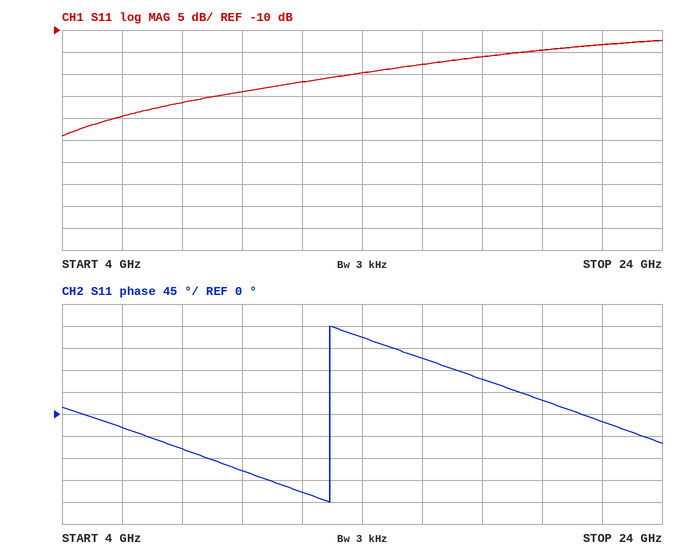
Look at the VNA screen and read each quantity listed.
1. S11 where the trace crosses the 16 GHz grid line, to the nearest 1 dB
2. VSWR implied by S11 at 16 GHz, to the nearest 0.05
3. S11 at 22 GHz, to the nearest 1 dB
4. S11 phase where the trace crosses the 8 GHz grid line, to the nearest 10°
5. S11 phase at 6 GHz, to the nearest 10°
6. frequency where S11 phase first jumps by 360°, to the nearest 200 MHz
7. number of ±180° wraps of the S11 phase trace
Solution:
-18 dB
1.30
-13 dB
-70°
-30°
13.0 GHz
1
